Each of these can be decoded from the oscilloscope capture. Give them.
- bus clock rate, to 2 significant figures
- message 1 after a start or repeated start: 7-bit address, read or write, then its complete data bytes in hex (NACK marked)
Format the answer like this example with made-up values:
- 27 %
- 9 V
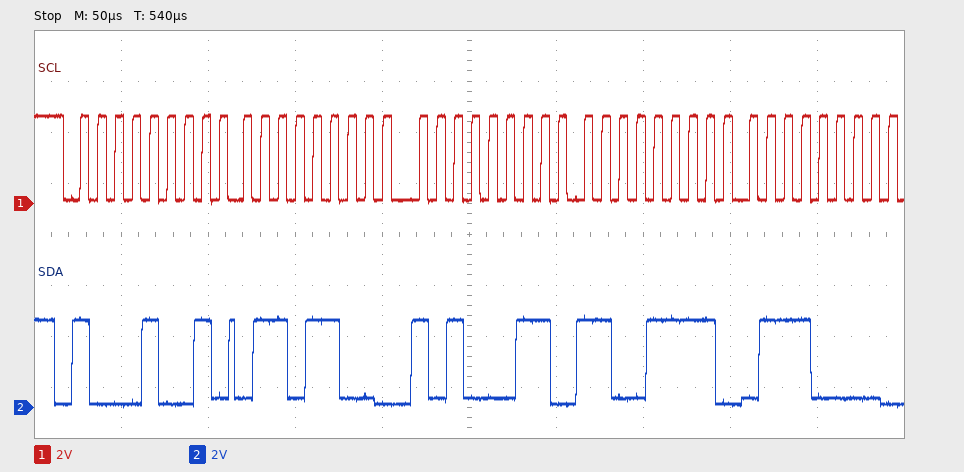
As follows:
- 100 kHz
- 0x44 read: 6C A3 CF 70
